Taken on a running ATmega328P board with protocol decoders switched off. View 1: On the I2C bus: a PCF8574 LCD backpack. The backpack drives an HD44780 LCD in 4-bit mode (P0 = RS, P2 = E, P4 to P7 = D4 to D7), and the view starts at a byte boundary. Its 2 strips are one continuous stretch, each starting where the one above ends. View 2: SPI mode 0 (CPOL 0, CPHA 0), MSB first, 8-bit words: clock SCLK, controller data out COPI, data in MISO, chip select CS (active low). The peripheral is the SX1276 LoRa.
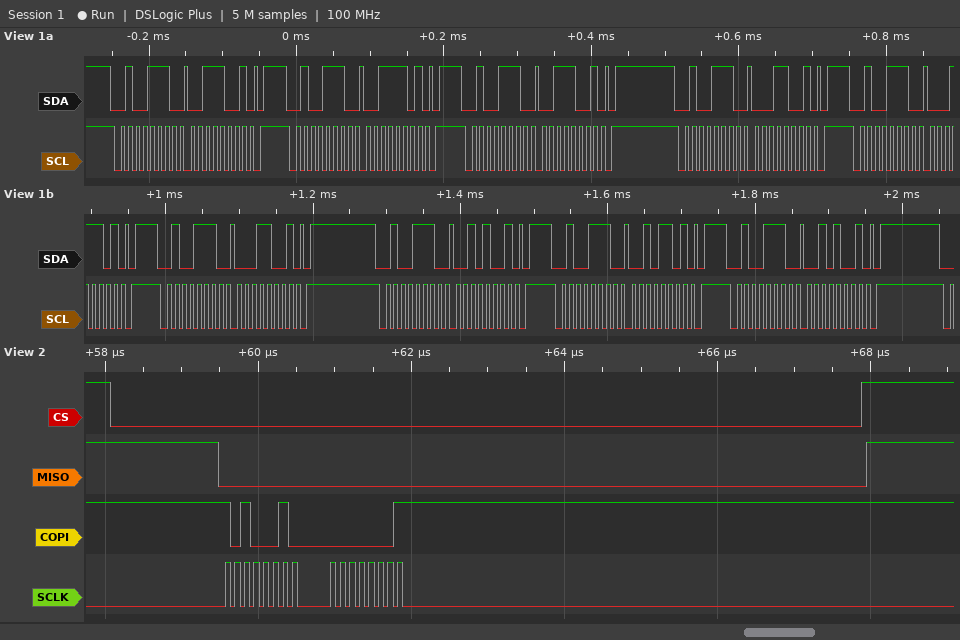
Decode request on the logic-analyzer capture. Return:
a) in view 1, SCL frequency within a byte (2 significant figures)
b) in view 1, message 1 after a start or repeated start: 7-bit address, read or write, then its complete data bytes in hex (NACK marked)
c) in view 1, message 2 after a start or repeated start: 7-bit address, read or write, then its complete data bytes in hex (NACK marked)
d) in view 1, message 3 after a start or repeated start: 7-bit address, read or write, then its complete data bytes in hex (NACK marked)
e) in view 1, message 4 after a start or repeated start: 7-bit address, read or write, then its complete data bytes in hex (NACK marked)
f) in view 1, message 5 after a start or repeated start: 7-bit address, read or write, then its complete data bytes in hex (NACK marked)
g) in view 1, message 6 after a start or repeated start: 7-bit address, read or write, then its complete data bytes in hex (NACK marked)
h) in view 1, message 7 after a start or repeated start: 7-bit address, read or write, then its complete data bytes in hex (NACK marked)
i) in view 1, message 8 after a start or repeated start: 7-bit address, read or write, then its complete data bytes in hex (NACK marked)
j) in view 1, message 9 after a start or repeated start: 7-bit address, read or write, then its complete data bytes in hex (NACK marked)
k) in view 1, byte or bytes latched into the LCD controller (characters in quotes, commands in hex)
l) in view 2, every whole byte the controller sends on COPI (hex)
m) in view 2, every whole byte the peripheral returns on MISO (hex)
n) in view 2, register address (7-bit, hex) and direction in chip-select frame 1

100 kHz
0x27 write: 39
0x27 write: 3D
0x27 write: 39
0x27 write: 19
0x27 write: 1D
0x27 write: 19
0x27 write: 29
0x27 write: 2D
0x27 write: 29
'1'
A2 01
00 00
0x22 write
